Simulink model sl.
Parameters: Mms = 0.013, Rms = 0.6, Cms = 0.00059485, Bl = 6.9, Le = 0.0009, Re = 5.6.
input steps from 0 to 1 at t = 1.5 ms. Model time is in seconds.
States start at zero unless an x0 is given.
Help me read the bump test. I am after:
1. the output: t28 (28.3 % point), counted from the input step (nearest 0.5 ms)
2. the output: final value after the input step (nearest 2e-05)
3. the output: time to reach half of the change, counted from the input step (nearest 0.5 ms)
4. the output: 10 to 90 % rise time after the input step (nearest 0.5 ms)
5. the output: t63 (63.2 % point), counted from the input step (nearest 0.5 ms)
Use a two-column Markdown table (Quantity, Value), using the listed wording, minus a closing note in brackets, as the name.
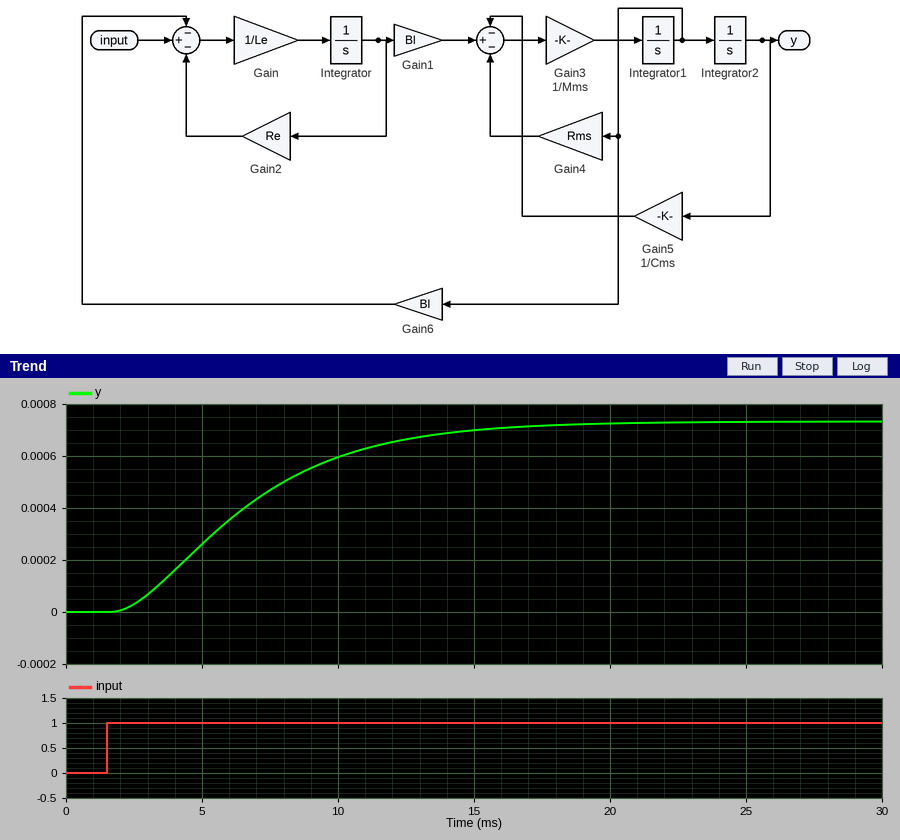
| Quantity | Value |
|---|---|
| the output: t28 (28.3 % point), counted from the input step | 3.0 ms |
| the output: final value after the input step | 0.00074 |
| the output: time to reach half of the change, counted from the input step | 4.5 ms |
| the output: 10 to 90 % rise time after the input step | 9.0 ms |
| the output: t63 (63.2 % point), counted from the input step | 6.0 ms |
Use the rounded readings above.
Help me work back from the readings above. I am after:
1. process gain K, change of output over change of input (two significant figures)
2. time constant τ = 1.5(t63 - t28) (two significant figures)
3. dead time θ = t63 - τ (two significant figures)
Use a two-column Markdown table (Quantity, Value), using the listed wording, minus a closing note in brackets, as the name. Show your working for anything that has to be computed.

| Quantity | Value |
|---|---|
| process gain K, change of output over change of input | (0.00074 - 0) / 1 = 0.00074 |
| time constant τ = 1.5(t63 - t28) | 1.5 × (6 - 3) = 4.5 ms |
| dead time θ = t63 - τ | 6 - 4.5 = 1.5 ms |
